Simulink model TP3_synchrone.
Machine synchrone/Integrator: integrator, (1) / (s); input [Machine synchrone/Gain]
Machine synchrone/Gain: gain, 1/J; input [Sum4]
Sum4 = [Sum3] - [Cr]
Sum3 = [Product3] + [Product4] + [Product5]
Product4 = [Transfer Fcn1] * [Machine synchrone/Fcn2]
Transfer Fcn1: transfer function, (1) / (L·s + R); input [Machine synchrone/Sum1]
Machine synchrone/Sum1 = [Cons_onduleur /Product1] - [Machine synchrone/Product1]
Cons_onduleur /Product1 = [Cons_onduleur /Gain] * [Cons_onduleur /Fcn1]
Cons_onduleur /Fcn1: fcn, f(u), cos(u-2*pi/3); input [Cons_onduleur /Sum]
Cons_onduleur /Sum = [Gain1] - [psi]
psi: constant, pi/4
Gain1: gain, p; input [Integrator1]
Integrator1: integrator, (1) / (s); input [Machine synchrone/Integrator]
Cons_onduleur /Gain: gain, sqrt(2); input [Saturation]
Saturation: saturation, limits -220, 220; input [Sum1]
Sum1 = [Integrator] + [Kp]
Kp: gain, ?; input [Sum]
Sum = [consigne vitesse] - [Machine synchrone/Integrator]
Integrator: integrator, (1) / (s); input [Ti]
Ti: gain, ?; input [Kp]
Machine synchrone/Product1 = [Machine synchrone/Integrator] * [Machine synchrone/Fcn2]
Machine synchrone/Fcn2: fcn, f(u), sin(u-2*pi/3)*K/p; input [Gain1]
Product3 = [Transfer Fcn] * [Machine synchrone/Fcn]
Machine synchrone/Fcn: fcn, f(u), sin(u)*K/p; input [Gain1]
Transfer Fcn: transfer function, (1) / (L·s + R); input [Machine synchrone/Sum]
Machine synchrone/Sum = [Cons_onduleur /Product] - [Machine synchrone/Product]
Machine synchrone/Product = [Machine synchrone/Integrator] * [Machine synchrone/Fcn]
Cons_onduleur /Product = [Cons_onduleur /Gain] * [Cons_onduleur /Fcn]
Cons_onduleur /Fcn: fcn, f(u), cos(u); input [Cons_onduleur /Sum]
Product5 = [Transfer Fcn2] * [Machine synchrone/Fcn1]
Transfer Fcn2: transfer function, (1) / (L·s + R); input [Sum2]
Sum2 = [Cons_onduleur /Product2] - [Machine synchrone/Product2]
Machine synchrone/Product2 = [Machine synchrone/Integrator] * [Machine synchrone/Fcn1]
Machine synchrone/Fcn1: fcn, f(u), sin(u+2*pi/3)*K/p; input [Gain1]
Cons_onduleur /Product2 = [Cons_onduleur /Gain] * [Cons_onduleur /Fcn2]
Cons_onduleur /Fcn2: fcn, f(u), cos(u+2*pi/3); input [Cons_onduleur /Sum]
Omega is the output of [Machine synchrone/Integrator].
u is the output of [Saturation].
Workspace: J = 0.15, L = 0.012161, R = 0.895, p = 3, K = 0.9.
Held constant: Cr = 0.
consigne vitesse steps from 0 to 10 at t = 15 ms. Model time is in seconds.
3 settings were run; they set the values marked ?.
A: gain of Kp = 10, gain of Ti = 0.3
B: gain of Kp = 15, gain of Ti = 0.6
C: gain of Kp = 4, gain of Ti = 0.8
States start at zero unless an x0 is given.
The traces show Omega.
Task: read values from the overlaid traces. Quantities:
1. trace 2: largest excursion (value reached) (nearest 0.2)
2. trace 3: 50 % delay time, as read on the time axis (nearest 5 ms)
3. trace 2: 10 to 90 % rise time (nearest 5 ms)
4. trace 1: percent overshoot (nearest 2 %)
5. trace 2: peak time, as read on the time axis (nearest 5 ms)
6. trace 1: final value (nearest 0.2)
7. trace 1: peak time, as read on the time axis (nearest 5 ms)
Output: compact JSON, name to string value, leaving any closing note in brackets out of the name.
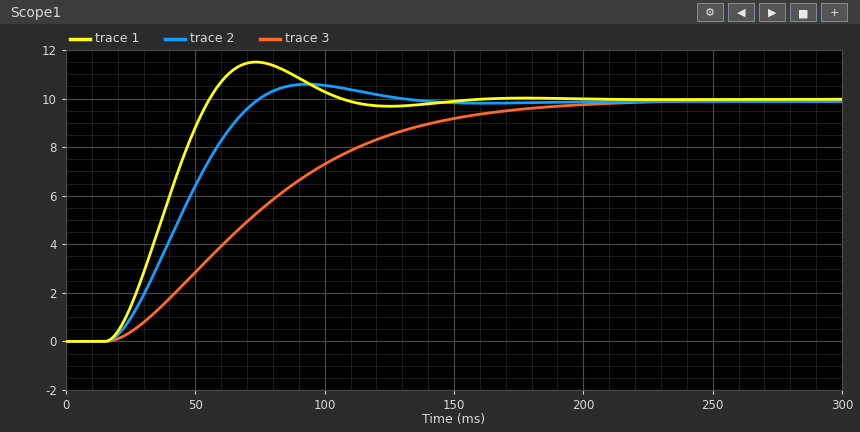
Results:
{"trace 2: largest excursion (value reached)": "10.6", "trace 3: 50 % delay time, as read on the time axis": "70 ms", "trace 2: 10 to 90 % rise time": "40 ms", "trace 1: percent overshoot": "16 %", "trace 2: peak time, as read on the time axis": "95 ms", "trace 1: final value": "10.0", "trace 1: peak time, as read on the time axis": "75 ms"}
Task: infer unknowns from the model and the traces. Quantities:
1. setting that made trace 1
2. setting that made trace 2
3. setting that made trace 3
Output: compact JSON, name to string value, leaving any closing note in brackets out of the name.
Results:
{"setting that made trace 1": "B", "setting that made trace 2": "A", "setting that made trace 3": "C"}
